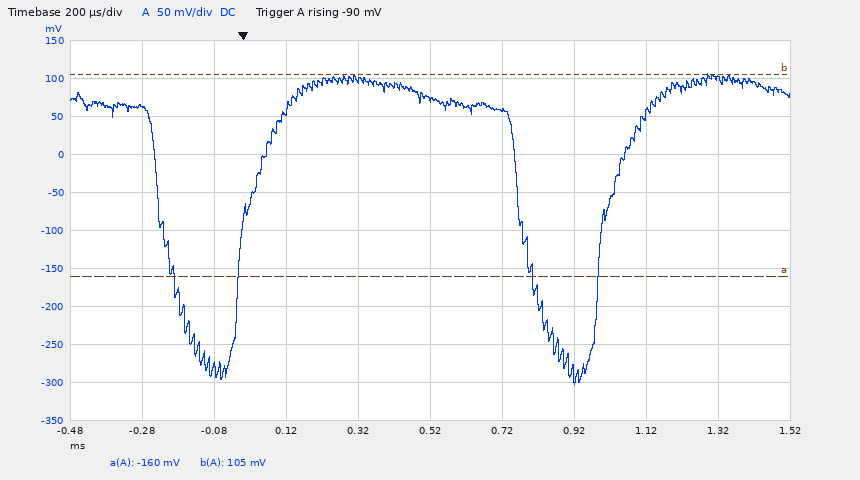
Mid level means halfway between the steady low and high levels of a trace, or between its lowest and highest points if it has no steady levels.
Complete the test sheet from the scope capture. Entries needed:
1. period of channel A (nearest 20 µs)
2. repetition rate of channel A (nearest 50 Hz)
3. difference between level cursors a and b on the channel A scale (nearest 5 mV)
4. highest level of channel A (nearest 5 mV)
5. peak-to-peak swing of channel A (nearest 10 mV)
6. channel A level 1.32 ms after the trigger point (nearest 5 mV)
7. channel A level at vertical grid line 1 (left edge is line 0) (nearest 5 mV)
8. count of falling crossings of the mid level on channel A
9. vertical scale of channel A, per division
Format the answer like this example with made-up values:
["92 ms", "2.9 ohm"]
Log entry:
["1.00 ms", "1.00 kHz", "265 mV", "105 mV", "410 mV", "100 mV", "65 mV", "2", "50 mV"]
